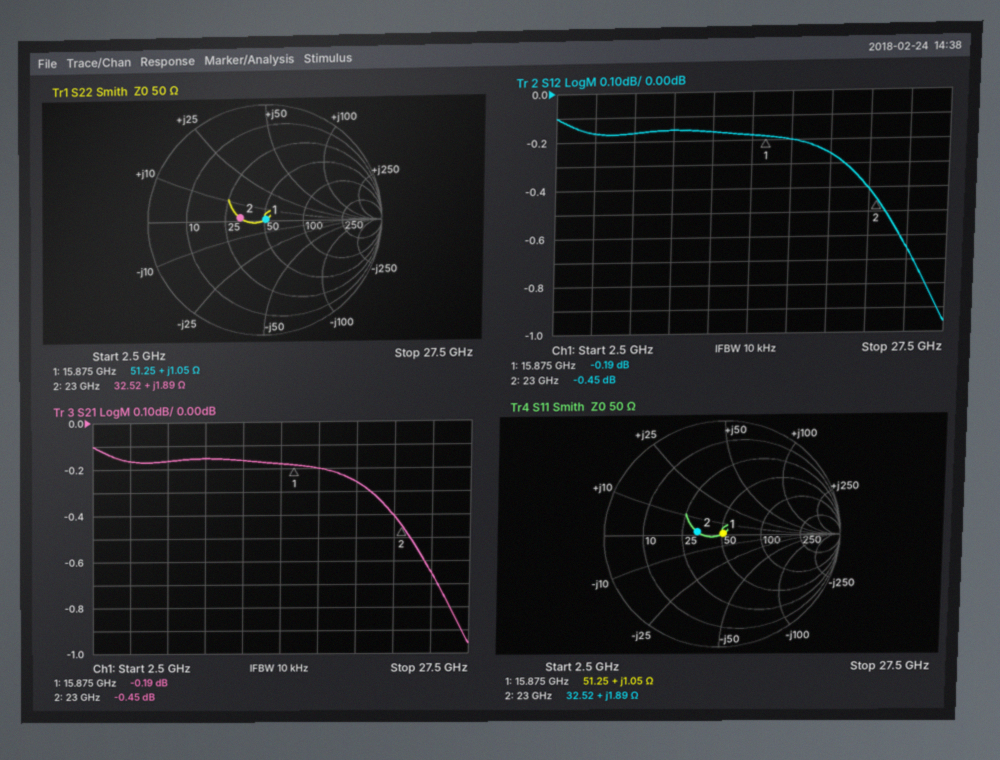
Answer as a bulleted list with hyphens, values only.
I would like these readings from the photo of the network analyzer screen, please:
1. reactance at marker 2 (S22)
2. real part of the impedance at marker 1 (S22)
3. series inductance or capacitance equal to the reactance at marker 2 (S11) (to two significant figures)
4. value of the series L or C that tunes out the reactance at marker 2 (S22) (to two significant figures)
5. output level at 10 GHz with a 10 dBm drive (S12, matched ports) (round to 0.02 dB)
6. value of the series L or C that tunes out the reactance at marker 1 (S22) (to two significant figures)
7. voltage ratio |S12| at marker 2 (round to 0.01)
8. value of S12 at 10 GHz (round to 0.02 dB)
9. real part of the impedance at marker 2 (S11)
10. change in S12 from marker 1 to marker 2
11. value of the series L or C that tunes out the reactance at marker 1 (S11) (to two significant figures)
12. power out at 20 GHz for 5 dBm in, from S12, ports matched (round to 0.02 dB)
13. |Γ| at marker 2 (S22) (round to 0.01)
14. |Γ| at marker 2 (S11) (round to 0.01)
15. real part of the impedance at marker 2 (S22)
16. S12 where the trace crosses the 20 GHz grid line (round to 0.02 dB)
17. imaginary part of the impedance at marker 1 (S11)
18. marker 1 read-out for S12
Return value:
- +1.89 Ω
- 51.25 Ω
- 13 pH
- 3.7 pF
- 9.84 dBm
- 9.5 pF
- 0.95
- -0.16 dB
- 32.52 Ω
- -0.26 dB
- 9.5 pF
- 4.74 dBm
- 0.21
- 0.21
- 32.52 Ω
- -0.26 dB
- +1.05 Ω
- -0.19 dB
